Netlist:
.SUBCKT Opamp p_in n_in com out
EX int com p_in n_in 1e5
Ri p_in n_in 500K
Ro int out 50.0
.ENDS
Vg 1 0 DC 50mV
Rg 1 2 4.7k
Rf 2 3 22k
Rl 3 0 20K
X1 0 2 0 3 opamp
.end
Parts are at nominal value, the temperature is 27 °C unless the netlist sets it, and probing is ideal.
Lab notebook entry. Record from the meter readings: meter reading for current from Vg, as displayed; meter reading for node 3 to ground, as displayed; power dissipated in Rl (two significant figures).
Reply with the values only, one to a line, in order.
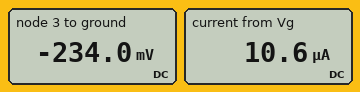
10.6 µA
-234.0 mV
2.7 µW
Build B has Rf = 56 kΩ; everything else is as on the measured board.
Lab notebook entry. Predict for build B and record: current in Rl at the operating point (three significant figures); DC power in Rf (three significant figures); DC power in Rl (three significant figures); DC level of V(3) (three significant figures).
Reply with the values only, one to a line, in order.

29.8 µA
6.34 µW
17.7 µW
-596 mV
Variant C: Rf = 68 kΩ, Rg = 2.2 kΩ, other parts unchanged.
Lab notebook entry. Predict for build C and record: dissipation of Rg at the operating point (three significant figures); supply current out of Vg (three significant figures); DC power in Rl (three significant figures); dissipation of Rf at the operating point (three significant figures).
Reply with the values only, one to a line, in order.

1.14 µW
22.7 µA
119 µW
35.1 µW
